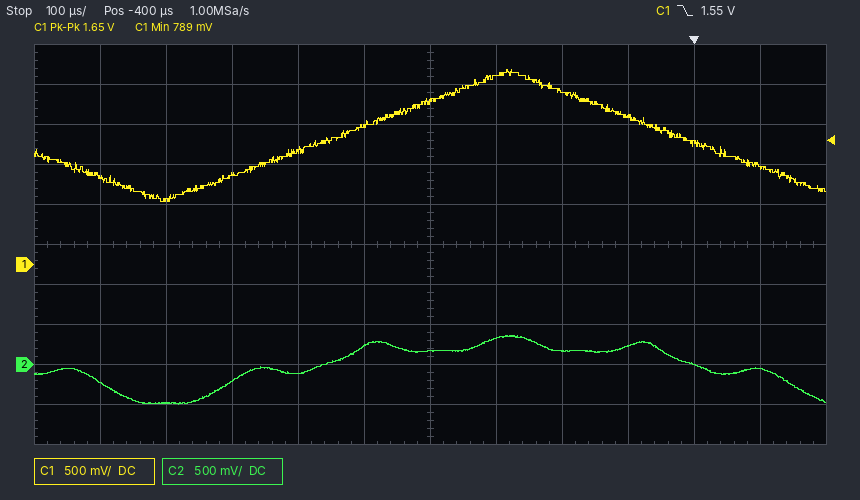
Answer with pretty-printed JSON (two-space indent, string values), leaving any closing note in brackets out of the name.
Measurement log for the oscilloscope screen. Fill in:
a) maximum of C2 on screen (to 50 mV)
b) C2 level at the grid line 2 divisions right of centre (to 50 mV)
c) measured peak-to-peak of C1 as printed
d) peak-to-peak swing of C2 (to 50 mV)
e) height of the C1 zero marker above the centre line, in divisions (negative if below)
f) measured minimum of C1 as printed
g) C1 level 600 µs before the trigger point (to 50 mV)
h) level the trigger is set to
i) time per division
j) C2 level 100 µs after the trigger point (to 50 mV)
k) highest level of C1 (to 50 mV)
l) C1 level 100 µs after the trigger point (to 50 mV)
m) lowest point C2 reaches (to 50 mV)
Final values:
{
  "maximum of C2 on screen": "350 mV",
  "C2 level at the grid line 2 divisions right of centre": "150 mV",
  "measured peak-to-peak of C1 as printed": "1.65 V",
  "peak-to-peak swing of C2": "850 mV",
  "height of the C1 zero marker above the centre line, in divisions": "-0.5 div",
  "measured minimum of C1 as printed": "789 mV",
  "C1 level 600 µs before the trigger point": "1.45 V",
  "level the trigger is set to": "1.55 V",
  "time per division": "100 µs",
  "C2 level 100 µs after the trigger point": "-50 mV",
  "highest level of C1": "2.45 V",
  "C1 level 100 µs after the trigger point": "1.25 V",
  "lowest point C2 reaches": "-500 mV"
}
